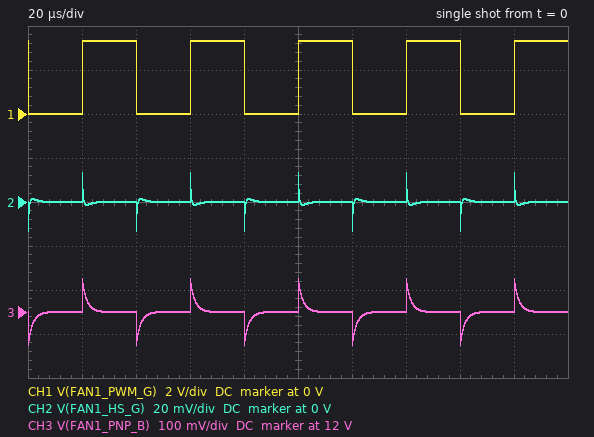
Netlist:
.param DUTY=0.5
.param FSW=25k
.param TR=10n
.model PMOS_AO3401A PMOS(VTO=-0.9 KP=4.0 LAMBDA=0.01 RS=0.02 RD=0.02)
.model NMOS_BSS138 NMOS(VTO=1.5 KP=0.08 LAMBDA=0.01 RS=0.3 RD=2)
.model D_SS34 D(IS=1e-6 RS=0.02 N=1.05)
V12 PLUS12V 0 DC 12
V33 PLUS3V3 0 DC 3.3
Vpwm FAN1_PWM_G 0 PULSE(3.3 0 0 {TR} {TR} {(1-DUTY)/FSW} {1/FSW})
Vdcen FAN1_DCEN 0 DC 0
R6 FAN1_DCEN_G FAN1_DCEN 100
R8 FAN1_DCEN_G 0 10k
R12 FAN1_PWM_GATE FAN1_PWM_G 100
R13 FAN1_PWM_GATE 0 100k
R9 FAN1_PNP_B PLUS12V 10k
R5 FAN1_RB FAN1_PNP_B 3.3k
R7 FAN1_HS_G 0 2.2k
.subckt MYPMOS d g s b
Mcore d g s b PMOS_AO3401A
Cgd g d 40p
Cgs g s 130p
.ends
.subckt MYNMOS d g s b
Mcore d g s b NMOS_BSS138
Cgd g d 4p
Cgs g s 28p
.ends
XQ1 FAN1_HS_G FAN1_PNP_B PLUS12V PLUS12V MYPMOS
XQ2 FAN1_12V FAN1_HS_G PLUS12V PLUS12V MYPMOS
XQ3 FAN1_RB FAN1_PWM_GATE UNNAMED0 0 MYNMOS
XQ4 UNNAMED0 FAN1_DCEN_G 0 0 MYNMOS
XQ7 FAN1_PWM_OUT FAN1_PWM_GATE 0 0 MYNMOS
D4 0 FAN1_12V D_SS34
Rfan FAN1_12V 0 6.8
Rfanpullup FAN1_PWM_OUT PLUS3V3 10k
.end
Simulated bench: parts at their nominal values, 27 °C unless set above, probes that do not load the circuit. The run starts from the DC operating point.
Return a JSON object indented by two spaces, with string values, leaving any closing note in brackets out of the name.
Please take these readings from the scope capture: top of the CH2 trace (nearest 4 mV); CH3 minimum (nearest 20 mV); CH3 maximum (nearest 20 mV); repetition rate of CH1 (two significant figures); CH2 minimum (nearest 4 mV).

{
  "top of the CH2 trace": "12 mV",
  "CH3 minimum": "11.92 V",
  "CH3 maximum": "12.08 V",
  "repetition rate of CH1": "25 kHz",
  "CH2 minimum": "-12 mV"
}
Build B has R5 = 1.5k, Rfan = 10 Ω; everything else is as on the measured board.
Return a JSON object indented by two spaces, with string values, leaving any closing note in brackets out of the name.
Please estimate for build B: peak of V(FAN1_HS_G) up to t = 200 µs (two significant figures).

{
  "peak of V(FAN1_HS_G) up to t = 200 µs": "14 mV"
}
